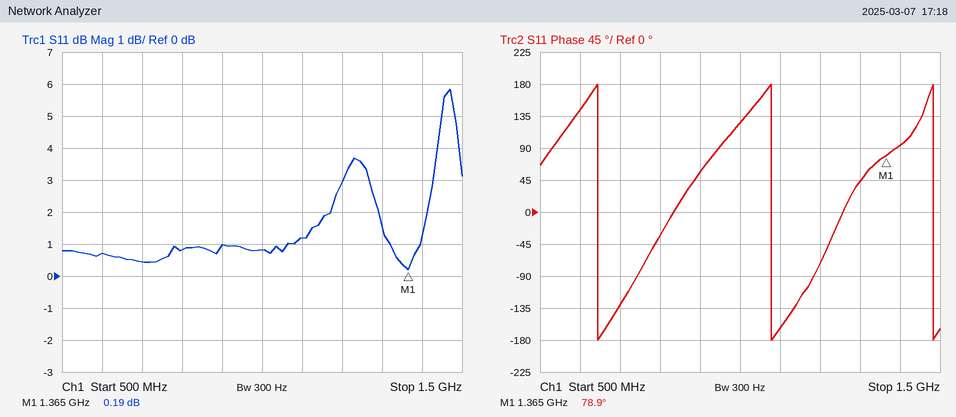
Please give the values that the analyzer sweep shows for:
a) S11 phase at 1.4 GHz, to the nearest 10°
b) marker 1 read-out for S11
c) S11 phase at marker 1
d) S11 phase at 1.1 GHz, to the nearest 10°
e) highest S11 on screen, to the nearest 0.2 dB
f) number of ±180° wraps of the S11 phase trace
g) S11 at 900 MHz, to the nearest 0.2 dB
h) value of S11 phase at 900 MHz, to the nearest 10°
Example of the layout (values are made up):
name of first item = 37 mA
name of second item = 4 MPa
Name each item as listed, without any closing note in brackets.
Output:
S11 phase at 1.4 GHz, to the nearest 10° = 90°
marker 1 read-out for S11 = 0.19 dB
S11 phase at marker 1 = 78.9°
S11 phase at 1.1 GHz, to the nearest 10° = -160°
highest S11 on screen, to the nearest 0.2 dB = 5.8 dB
number of ±180° wraps of the S11 phase trace = 3
S11 at 900 MHz, to the nearest 0.2 dB = 1.0 dB
value of S11 phase at 900 MHz, to the nearest 10° = 60°
